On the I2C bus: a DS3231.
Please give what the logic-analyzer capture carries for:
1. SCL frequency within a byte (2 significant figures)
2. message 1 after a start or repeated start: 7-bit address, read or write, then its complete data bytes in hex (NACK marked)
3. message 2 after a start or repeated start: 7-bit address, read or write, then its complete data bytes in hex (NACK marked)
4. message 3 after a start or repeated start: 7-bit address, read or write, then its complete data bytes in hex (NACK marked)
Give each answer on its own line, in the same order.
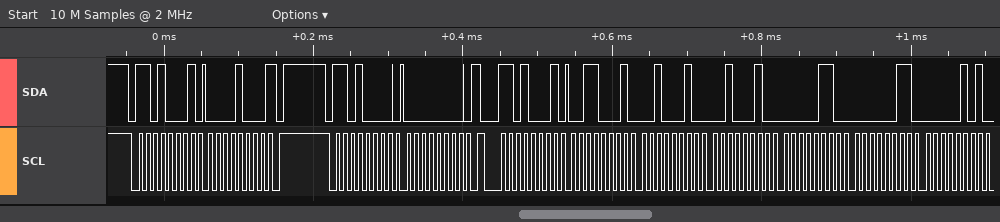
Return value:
100 kHz
0x68 read: 08 NACK
0x68 write: 00
0x68 read: 31 22 22 06 03 05
